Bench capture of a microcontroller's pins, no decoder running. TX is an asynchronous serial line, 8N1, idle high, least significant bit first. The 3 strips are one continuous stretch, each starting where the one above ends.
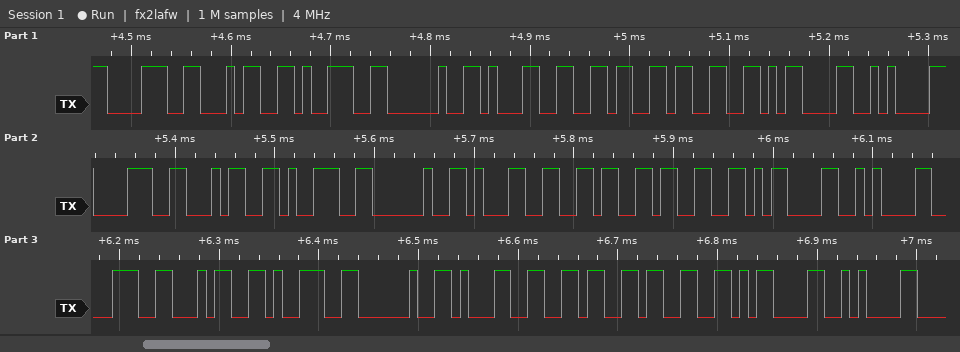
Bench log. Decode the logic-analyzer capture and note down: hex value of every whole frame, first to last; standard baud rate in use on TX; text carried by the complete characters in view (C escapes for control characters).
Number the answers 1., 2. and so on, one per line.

1. 38 34 39 20 31 36 33 0D 0A 38 34 39 20 31 36 33 0D 0A 38 34 39 20 31 36 33 0D 0A
2. 115200 baud
3. "849 163\r\n849 163\r\n849 163\r\n"
